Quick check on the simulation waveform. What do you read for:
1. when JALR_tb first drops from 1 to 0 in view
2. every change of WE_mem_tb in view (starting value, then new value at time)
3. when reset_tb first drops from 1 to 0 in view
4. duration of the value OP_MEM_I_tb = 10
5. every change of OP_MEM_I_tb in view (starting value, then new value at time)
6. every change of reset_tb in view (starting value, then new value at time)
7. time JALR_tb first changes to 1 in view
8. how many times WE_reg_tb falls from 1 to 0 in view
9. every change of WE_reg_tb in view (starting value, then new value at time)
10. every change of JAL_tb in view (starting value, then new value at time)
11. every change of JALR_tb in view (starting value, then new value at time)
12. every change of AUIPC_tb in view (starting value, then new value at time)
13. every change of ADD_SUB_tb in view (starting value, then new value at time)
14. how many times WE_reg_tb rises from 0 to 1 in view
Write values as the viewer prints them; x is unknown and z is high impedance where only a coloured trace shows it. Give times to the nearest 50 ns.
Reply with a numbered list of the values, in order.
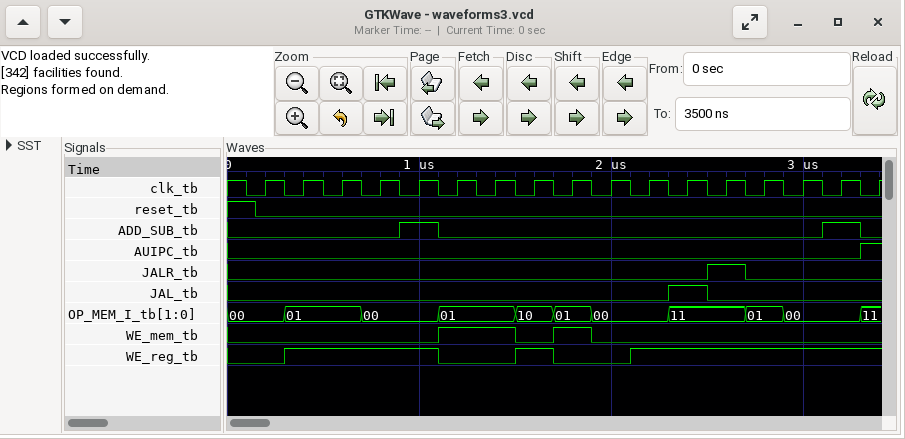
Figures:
1. 2700 ns
2. 0, 1 at 1100 ns, 0 at 1500 ns, 1 at 1700 ns, 0 at 1900 ns
3. 150 ns
4. 200 ns
5. 00, 01 at 300 ns, 00 at 700 ns, 01 at 1100 ns, 10 at 1500 ns, 01 at 1700 ns, 00 at 1900 ns, 11 at 2300 ns, 01 at 2700 ns, 00 at 2900 ns, 11 at 3300 ns
6. 1, 0 at 150 ns
7. 2500 ns
8. 2
9. 0, 1 at 300 ns, 0 at 1100 ns, 1 at 1500 ns, 0 at 1700 ns, 1 at 2100 ns
10. 0, 1 at 2300 ns, 0 at 2500 ns
11. 0, 1 at 2500 ns, 0 at 2700 ns
12. 0, 1 at 3300 ns
13. 0, 1 at 900 ns, 0 at 1100 ns, 1 at 3100 ns, 0 at 3300 ns
14. 3
